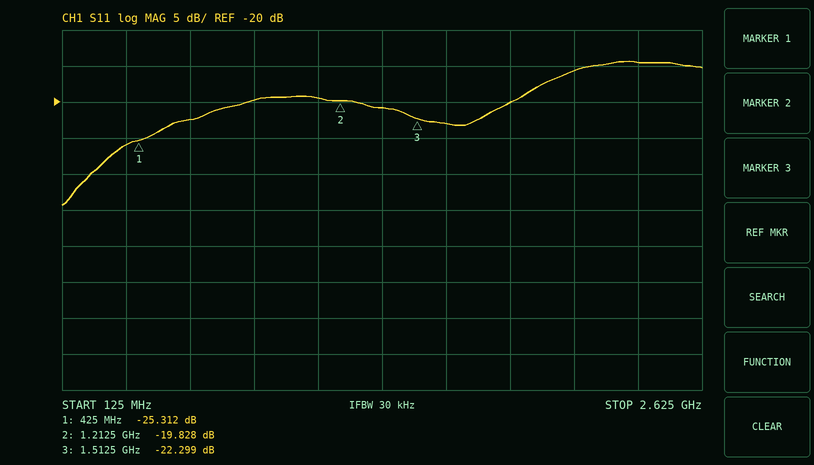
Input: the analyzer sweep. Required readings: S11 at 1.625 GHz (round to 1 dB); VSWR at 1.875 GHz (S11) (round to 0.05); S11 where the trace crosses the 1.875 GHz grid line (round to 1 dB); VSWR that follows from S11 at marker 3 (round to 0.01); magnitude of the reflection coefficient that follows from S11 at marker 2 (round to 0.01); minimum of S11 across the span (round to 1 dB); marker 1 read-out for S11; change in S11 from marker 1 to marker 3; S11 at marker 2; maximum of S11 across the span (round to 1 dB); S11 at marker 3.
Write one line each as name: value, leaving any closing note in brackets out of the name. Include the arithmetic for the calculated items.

S11 at 1.625 GHz: -23 dB
VSWR at 1.875 GHz (S11): |Γ| = 10^(-20/20) = 0.1000; VSWR = (1 + 0.1000)/(1 − 0.1000) ≈ 1.22, so 1.20 to the nearest 0.05
S11 where the trace crosses the 1.875 GHz grid line: -20 dB
VSWR that follows from S11 at marker 3: (1 + 0.0767)/(1 − 0.0767) ≈ 1.17
magnitude of the reflection coefficient that follows from S11 at marker 2: 10^(-19.828/20) ≈ 0.10
minimum of S11 across the span: -34 dB
marker 1 read-out for S11: -25.312 dB
change in S11 from marker 1 to marker 3: -22.299 − (-25.312) = 3.013 dB
S11 at marker 2: -19.828 dB
maximum of S11 across the span: -14 dB
S11 at marker 3: -22.299 dB
